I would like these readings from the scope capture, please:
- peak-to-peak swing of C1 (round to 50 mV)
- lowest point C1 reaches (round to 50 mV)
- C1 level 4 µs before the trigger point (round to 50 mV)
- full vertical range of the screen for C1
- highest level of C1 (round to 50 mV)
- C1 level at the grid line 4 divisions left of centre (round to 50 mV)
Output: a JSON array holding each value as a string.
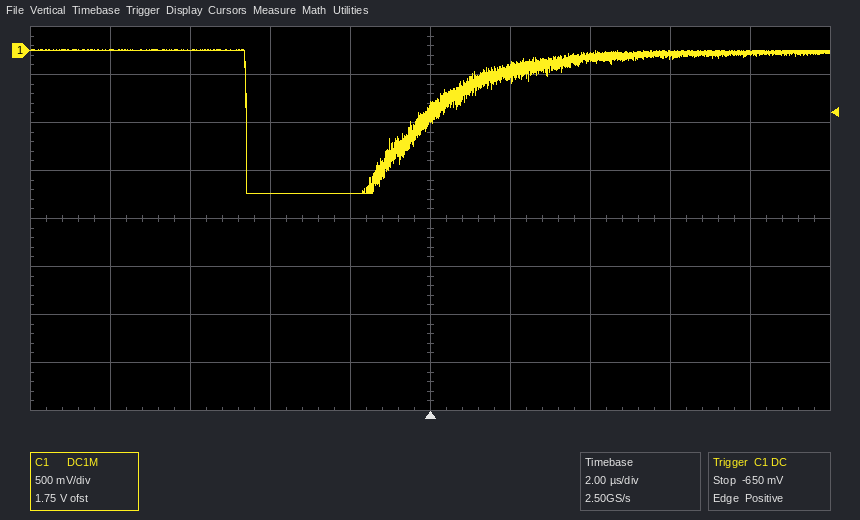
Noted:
["1.50 V", "-1.50 V", "-1.50 V", "4 V", "0 mV", "0 mV"]
